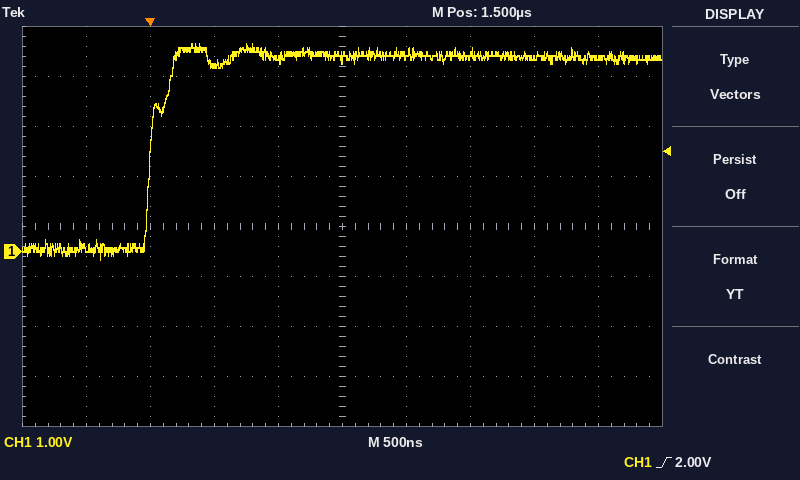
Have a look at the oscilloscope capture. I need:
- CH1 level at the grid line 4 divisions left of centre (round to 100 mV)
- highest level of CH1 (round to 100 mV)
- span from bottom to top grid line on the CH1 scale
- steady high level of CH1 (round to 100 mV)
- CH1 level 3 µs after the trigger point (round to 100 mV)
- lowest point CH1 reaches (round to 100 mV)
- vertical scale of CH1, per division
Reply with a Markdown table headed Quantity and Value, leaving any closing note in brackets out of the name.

| Quantity | Value |
|---|---|
| CH1 level at the grid line 4 divisions left of centre | 100 mV |
| highest level of CH1 | 4.2 V |
| span from bottom to top grid line on the CH1 scale | 8 V |
| steady high level of CH1 | 3.9 V |
| CH1 level 3 µs after the trigger point | 3.9 V |
| lowest point CH1 reaches | -200 mV |
| vertical scale of CH1, per division | 1 V |
